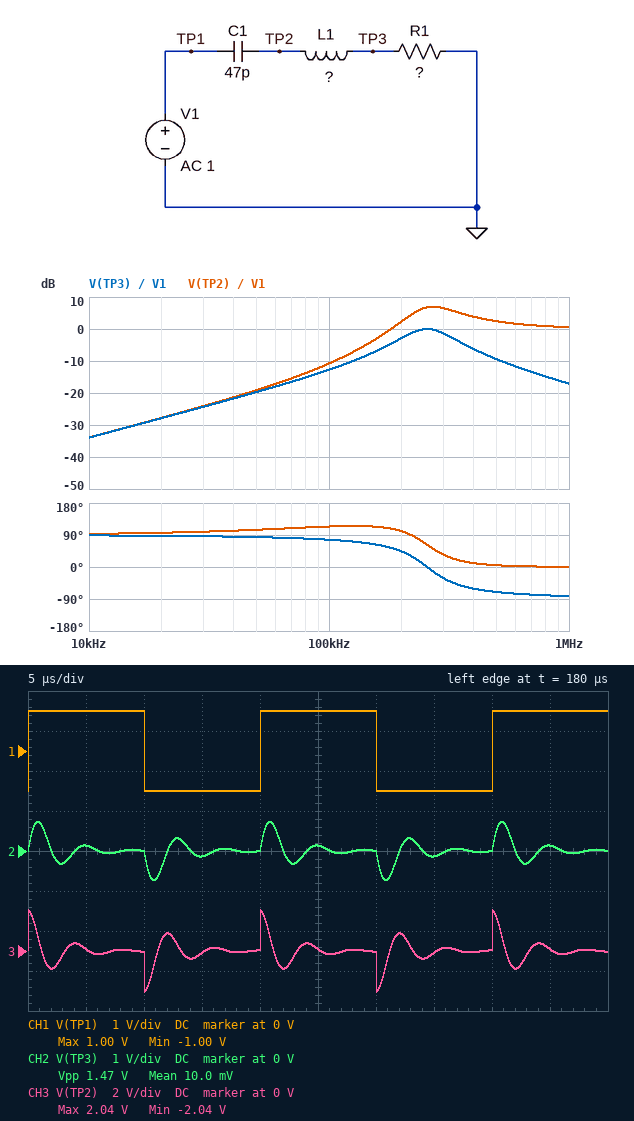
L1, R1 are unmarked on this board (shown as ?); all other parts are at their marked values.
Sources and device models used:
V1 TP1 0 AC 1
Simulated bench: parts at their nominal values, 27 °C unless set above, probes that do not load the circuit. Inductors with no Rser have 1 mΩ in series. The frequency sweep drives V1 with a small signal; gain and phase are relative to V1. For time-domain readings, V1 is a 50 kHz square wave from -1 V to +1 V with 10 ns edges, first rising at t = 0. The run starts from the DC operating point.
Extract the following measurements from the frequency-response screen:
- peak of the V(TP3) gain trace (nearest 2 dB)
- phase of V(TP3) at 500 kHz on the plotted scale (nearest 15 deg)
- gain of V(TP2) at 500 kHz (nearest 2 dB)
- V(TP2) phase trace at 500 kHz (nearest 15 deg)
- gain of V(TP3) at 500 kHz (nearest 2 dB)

0 dB
-75 deg
2 dB
0 deg
-10 dB
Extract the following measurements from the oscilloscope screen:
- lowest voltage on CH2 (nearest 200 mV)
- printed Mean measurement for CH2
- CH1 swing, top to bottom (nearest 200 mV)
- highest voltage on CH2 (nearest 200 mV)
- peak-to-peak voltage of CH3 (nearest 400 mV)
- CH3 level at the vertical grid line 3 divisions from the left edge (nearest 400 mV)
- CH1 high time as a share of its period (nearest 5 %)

-800 mV
10.0 mV
2.0 V
800 mV
4.0 V
0 V
50 %
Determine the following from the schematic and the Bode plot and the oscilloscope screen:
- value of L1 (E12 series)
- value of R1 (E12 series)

8.2 mH
6.8 kΩ
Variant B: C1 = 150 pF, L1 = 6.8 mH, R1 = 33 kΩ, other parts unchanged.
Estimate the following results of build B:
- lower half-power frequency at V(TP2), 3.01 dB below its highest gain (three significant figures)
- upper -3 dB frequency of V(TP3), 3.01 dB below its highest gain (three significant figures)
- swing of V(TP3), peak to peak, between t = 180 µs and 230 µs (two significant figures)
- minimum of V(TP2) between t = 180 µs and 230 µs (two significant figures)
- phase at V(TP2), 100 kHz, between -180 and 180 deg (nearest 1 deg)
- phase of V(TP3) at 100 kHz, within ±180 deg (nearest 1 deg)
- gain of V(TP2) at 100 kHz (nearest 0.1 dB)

32.8 kHz
803 kHz
3.2 V
-1.8 V
18 deg
11 deg
-0.1 dB
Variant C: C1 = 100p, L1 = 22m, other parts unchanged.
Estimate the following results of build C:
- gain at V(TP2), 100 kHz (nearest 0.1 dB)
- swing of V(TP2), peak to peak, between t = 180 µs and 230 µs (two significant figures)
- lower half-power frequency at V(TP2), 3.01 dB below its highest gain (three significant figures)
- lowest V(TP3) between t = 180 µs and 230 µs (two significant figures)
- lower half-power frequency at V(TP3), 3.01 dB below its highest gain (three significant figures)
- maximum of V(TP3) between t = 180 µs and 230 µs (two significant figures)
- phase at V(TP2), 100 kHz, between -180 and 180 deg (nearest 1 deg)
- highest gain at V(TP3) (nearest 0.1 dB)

6.7 dB
3.3 V
91.4 kHz
-550 mV
85.5 kHz
550 mV
81 deg
0 dB
